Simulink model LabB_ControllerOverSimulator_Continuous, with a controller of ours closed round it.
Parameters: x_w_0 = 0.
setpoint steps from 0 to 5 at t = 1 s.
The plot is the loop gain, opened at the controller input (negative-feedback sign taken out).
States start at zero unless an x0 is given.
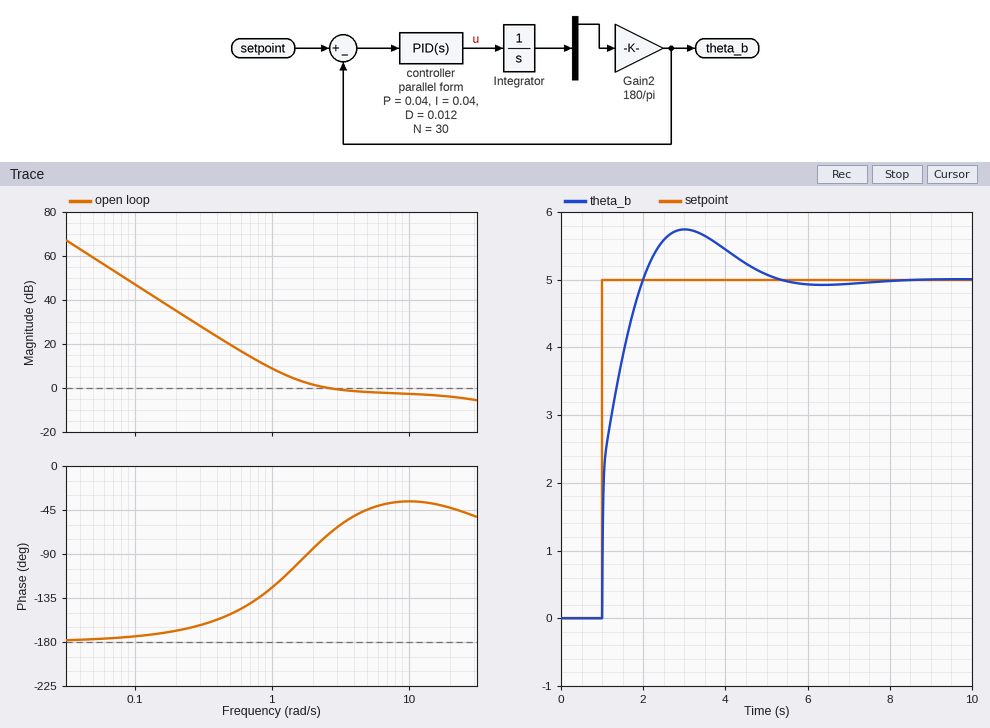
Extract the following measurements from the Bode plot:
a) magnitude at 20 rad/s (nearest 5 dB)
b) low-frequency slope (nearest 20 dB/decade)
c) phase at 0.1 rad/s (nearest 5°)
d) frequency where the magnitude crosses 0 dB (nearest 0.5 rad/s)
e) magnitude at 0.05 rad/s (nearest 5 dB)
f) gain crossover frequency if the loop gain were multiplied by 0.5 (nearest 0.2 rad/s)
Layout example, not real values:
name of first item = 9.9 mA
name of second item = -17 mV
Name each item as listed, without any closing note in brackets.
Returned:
magnitude at 20 rad/s = -5 dB
low-frequency slope = -40 dB/decade
phase at 0.1 rad/s = -175°
frequency where the magnitude crosses 0 dB = 2.5 rad/s
magnitude at 0.05 rad/s = 60 dB
gain crossover frequency if the loop gain were multiplied by 0.5 = 1.2 rad/s
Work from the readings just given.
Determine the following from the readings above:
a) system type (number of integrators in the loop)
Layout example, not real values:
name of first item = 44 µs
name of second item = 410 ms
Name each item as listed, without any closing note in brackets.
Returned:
system type = 2
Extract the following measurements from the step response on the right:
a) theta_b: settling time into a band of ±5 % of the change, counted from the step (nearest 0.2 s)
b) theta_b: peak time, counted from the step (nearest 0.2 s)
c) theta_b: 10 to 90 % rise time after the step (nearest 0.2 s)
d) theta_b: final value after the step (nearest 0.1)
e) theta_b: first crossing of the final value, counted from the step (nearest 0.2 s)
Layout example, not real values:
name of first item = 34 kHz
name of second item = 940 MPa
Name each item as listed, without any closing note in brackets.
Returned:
theta_b: settling time into a band of ±5 % of the change, counted from the step = 3.4 s
theta_b: peak time, counted from the step = 2.0 s
theta_b: 10 to 90 % rise time after the step = 0.8 s
theta_b: final value after the step = 5.0
theta_b: first crossing of the final value, counted from the step = 1.0 s
